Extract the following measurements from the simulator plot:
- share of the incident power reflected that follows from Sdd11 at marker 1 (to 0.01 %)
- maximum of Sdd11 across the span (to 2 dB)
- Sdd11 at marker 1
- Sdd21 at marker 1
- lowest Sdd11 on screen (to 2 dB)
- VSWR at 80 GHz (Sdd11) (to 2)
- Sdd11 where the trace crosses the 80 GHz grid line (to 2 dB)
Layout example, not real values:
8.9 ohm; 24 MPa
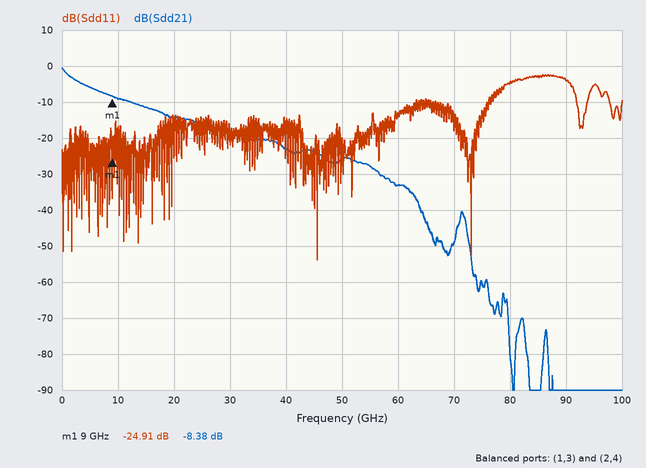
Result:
0.32 %; -2 dB; -24.91 dB; -8.38 dB; -54 dB; 4; -4 dB
